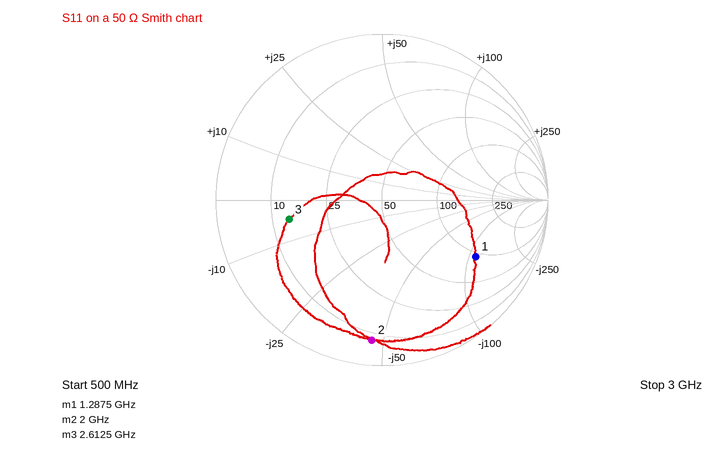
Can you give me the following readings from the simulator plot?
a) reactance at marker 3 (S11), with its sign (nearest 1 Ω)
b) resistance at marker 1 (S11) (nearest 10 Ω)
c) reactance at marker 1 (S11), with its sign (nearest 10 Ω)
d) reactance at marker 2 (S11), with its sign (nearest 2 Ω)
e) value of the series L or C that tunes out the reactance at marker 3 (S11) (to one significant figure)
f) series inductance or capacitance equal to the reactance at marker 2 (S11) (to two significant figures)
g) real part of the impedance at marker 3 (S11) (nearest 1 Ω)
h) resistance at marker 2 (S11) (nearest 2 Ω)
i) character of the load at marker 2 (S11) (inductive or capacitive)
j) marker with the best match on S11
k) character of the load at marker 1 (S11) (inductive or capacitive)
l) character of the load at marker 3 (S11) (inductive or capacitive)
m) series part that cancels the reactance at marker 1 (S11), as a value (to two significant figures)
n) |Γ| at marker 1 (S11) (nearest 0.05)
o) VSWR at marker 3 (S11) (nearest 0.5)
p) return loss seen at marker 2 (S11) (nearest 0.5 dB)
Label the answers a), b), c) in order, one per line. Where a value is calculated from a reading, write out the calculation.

a) -5 Ω
b) 90 Ω
c) -110 Ω
d) -46 Ω
e) L = 5 Ω/(2π × 2.6125 GHz) ≈ 305 pH, so 300 pH to one significant figure
f) C = 1/(2π × 2 GHz × 46 Ω) ≈ 1.7 pF
g) 14 Ω
h) 8 Ω
i) capacitive
j) marker 3
k) capacitive
l) capacitive
m) L = 110 Ω/(2π × 1.2875 GHz) ≈ 14 nH
n) 0.65
o) 3.5
p) 1.5 dB
